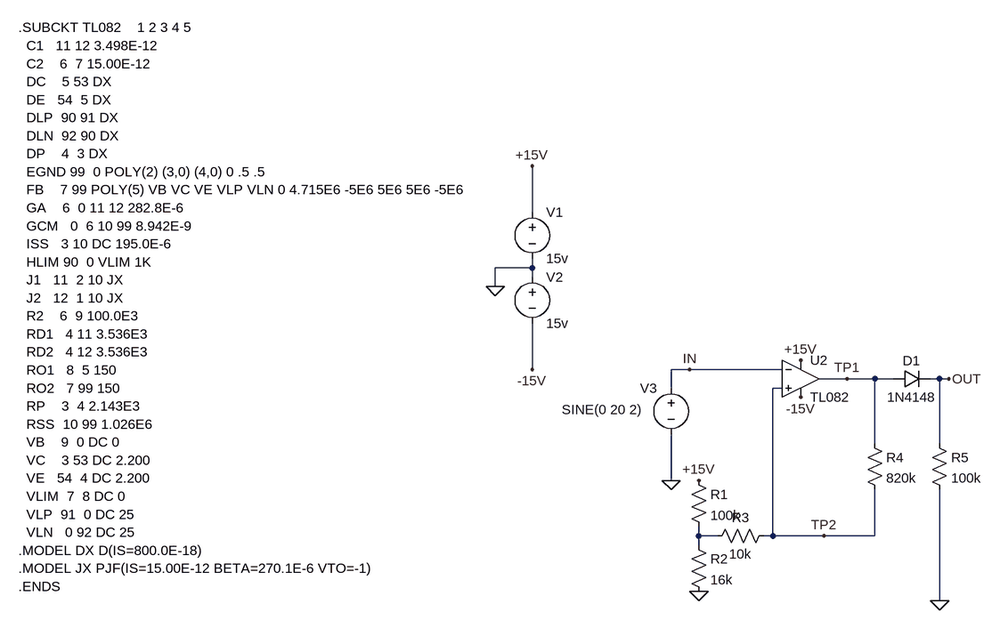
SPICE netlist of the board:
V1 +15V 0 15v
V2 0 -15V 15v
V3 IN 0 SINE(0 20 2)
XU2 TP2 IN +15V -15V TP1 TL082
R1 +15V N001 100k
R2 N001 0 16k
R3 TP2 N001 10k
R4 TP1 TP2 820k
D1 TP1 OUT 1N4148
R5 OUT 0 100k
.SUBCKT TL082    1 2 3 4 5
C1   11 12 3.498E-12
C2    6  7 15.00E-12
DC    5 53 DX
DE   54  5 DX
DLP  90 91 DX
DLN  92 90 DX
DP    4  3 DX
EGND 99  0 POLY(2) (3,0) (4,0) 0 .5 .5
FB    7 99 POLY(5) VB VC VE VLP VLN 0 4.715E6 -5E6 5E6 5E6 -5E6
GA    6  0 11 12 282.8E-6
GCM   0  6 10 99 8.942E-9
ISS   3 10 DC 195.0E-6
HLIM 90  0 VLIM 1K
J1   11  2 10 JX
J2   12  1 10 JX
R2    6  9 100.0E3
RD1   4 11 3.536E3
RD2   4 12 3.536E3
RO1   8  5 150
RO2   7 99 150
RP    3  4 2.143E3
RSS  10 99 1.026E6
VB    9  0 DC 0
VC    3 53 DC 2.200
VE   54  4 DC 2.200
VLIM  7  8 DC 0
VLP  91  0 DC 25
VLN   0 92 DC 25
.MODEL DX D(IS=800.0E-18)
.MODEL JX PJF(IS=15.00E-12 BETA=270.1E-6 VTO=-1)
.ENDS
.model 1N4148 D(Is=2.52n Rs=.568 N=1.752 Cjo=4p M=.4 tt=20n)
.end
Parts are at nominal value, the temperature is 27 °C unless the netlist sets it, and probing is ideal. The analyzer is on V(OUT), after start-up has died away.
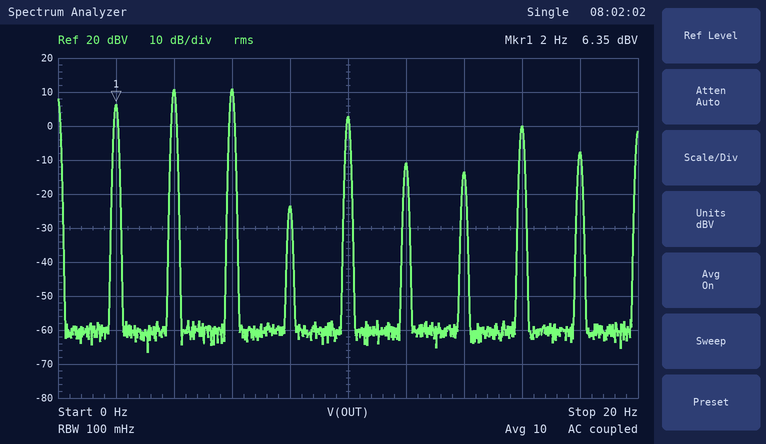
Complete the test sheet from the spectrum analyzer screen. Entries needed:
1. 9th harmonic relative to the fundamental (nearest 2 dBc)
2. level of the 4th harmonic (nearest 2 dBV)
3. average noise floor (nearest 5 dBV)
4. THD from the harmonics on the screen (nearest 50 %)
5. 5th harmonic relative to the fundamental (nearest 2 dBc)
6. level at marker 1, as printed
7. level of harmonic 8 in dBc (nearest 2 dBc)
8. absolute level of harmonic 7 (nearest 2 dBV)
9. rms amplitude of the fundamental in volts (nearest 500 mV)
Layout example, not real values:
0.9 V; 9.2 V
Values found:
-14 dBc; -24 dBV; -60 dBV; 250 %; -4 dBc; 6.35 dBV; -6 dBc; -14 dBV; 2.0 V
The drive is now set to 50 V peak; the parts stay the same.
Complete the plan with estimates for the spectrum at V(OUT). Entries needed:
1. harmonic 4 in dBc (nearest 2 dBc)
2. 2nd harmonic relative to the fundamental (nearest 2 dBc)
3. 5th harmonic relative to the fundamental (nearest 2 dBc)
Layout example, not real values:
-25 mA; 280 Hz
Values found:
16 dBc; 16 dBc; 12 dBc
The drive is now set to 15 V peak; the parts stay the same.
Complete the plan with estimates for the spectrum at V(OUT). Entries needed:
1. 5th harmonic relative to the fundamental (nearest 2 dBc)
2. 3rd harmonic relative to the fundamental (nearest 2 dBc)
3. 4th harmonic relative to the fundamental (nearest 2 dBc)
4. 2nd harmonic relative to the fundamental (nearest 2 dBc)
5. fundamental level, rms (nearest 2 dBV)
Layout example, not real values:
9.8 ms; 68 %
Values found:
-16 dBc; -10 dBc; -18 dBc; -18 dBc; 16 dBV
